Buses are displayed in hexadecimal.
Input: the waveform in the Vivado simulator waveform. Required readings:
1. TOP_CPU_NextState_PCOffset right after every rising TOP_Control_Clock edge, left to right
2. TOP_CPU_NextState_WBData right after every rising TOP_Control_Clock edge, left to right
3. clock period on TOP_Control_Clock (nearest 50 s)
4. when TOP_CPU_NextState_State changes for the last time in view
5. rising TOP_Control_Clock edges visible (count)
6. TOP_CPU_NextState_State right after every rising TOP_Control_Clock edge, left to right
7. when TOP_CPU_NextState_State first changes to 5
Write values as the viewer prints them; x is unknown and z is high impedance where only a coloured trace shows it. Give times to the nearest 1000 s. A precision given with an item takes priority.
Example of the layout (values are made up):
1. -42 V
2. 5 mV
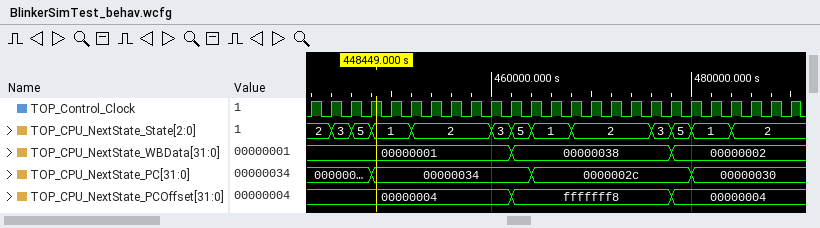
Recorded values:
1. 00000004, 00000004, 00000004, 00000004, 00000004, 00000004, 00000004, 00000004, 00000004, 00000004, fffffff8, fffffff8, fffffff8, fffffff8, fffffff8, fffffff8, fffffff8, fffffff8, 00000004, 00000004, 00000004, 00000004, 00000004, 00000004, 00000004
2. 00000001, 00000001, 00000001, 00000001, 00000001, 00000001, 00000001, 00000001, 00000001, 00000001, 00000038, 00000038, 00000038, 00000038, 00000038, 00000038, 00000038, 00000038, 00000002, 00000002, 00000002, 00000002, 00000002, 00000002, 00000002
3. 2000 s
4. 484000 s
5. 25
6. 2, 3, 5, 1, 1, 2, 2, 2, 2, 3, 5, 1, 1, 2, 2, 2, 2, 3, 5, 1, 1, 2, 2, 2, 2
7. 446000 s
